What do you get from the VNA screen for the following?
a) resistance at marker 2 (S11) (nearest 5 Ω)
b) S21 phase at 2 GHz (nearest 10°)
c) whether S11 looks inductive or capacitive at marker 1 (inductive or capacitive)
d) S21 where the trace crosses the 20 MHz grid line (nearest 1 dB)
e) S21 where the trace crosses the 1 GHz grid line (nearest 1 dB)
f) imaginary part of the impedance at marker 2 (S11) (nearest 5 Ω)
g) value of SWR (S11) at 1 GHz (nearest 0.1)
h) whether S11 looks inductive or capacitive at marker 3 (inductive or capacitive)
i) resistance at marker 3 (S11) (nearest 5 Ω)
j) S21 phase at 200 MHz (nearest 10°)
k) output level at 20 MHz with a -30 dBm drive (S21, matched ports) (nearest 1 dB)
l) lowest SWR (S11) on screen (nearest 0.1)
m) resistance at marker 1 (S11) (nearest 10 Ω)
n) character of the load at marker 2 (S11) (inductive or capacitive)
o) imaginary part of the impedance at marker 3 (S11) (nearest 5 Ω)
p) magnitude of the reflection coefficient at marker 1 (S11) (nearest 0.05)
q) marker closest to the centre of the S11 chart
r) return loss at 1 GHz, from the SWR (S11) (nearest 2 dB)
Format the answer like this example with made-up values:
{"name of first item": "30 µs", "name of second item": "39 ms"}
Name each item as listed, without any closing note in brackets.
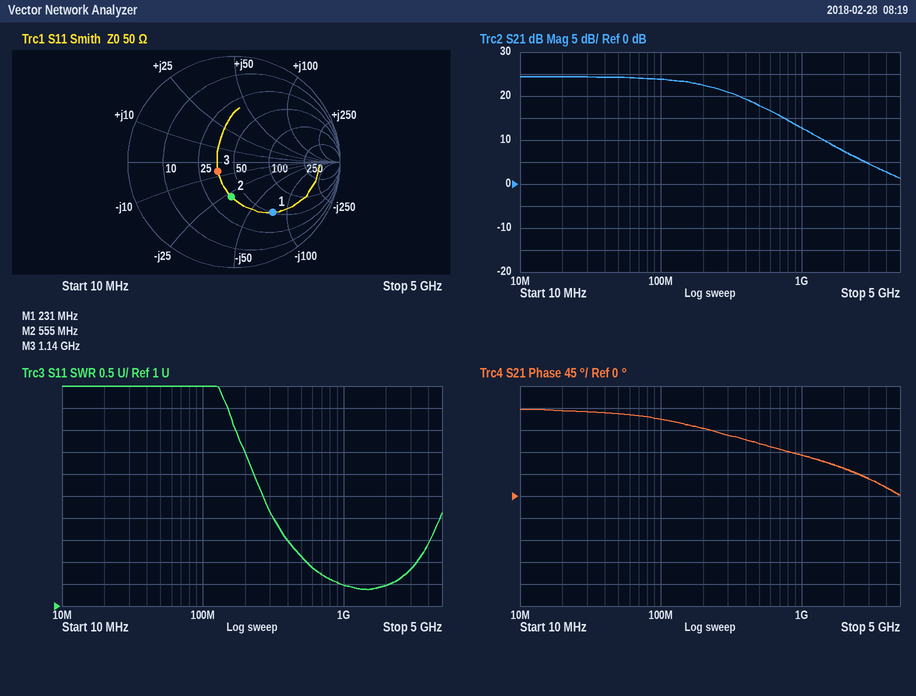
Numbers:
{"resistance at marker 2 (S11)": "40 Ω", "S21 phase at 2 GHz": "60°", "whether S11 looks inductive or capacitive at marker 1": "capacitive", "S21 where the trace crosses the 20 MHz grid line": "24 dB", "S21 where the trace crosses the 1 GHz grid line": "13 dB", "imaginary part of the impedance at marker 2 (S11)": "-30 Ω", "value of SWR (S11) at 1 GHz": "1.5", "whether S11 looks inductive or capacitive at marker 3": "capacitive", "resistance at marker 3 (S11)": "35 Ω", "S21 phase at 200 MHz": "140°", "output level at 20 MHz with a -30 dBm drive (S21, matched ports)": "-6 dBm", "lowest SWR (S11) on screen": "1.4", "resistance at marker 1 (S11)": "50 Ω", "character of the load at marker 2 (S11)": "capacitive", "imaginary part of the impedance at marker 3 (S11)": "-5 Ω", "magnitude of the reflection coefficient at marker 1 (S11)": "0.60", "marker closest to the centre of the S11 chart": "marker 3", "return loss at 1 GHz, from the SWR (S11)": "14 dB"}
